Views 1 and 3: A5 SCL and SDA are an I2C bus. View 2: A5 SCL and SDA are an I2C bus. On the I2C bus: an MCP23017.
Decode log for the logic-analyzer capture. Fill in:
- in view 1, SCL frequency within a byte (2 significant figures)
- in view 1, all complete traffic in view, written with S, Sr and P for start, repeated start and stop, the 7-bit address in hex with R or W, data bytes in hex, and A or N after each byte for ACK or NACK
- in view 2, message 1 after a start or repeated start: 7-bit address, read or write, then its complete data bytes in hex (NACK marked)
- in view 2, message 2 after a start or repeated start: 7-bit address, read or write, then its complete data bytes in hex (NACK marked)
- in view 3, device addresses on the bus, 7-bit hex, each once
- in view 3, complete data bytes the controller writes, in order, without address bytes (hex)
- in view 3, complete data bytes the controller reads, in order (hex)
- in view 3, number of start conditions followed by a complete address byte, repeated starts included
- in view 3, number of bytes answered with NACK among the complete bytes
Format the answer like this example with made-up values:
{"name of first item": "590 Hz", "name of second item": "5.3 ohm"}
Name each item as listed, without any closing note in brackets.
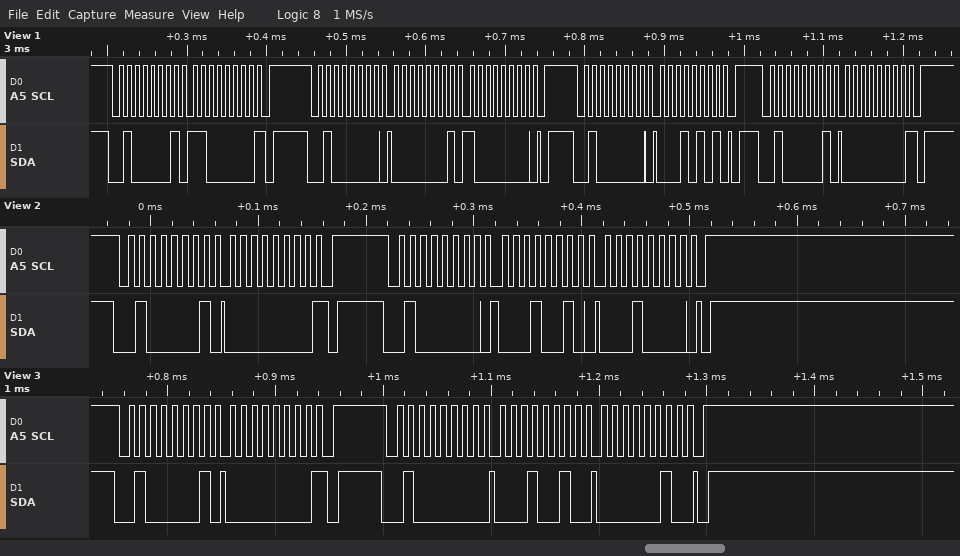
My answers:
{"in view 1, SCL frequency within a byte": "100 kHz", "in view 1, all complete traffic in view, written with S, Sr and P for start, repeated start and stop, the 7-bit address in hex with R or W, data bytes in hex, and A or N after each byte for ACK or NACK": "S 20R A C0 N P S 20W A 01 A 80 A P S 20W A 15 A P S 20R A 00 N P", "in view 2, message 1 after a start or repeated start: 7-bit address, read or write, then its complete data bytes in hex": "0x20 read: 00 NACK", "in view 2, message 2 after a start or repeated start: 7-bit address, read or write, then its complete data bytes in hex": "0x20 write: 12 10", "in view 3, device addresses on the bus, 7-bit hex, each once": "0x20", "in view 3, complete data bytes the controller writes, in order, without address bytes": "12 02", "in view 3, complete data bytes the controller reads, in order": "00", "in view 3, number of start conditions followed by a complete address byte, repeated starts included": "2", "in view 3, number of bytes answered with NACK among the complete bytes": "1"}
